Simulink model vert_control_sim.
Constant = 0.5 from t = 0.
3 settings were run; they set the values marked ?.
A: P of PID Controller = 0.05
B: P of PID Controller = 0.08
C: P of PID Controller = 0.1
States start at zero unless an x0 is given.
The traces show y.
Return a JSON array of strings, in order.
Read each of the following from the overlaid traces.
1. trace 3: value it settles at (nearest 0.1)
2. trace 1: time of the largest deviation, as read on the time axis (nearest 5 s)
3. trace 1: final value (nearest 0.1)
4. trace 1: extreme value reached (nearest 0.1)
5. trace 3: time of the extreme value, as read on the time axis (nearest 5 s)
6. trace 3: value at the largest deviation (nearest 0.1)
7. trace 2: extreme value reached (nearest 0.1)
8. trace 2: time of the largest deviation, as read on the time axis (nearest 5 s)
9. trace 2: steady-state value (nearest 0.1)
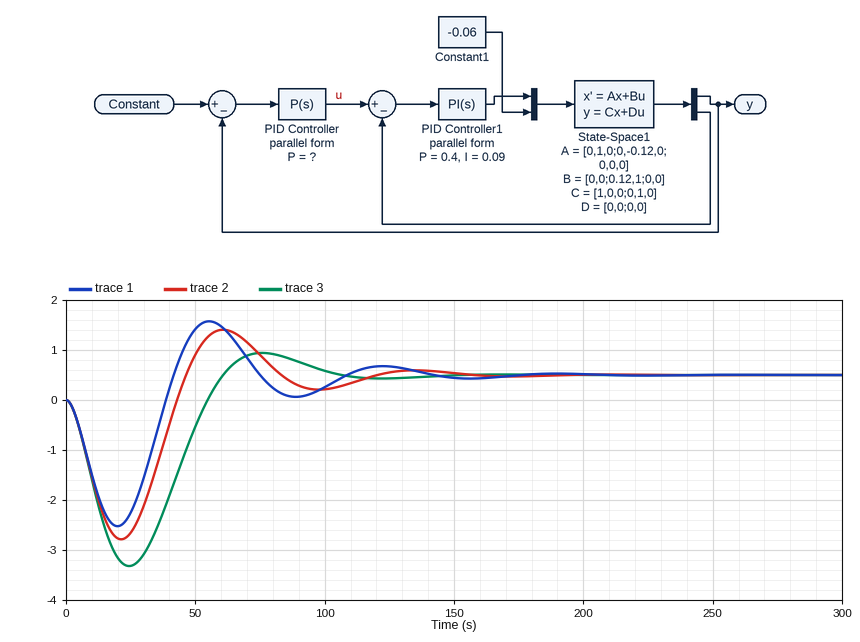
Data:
["0.5", "20 s", "0.5", "-2.5", "25 s", "-3.3", "-2.8", "20 s", "0.5"]
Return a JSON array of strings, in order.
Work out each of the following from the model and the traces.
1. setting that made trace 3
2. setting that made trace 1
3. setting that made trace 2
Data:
["A", "C", "B"]
